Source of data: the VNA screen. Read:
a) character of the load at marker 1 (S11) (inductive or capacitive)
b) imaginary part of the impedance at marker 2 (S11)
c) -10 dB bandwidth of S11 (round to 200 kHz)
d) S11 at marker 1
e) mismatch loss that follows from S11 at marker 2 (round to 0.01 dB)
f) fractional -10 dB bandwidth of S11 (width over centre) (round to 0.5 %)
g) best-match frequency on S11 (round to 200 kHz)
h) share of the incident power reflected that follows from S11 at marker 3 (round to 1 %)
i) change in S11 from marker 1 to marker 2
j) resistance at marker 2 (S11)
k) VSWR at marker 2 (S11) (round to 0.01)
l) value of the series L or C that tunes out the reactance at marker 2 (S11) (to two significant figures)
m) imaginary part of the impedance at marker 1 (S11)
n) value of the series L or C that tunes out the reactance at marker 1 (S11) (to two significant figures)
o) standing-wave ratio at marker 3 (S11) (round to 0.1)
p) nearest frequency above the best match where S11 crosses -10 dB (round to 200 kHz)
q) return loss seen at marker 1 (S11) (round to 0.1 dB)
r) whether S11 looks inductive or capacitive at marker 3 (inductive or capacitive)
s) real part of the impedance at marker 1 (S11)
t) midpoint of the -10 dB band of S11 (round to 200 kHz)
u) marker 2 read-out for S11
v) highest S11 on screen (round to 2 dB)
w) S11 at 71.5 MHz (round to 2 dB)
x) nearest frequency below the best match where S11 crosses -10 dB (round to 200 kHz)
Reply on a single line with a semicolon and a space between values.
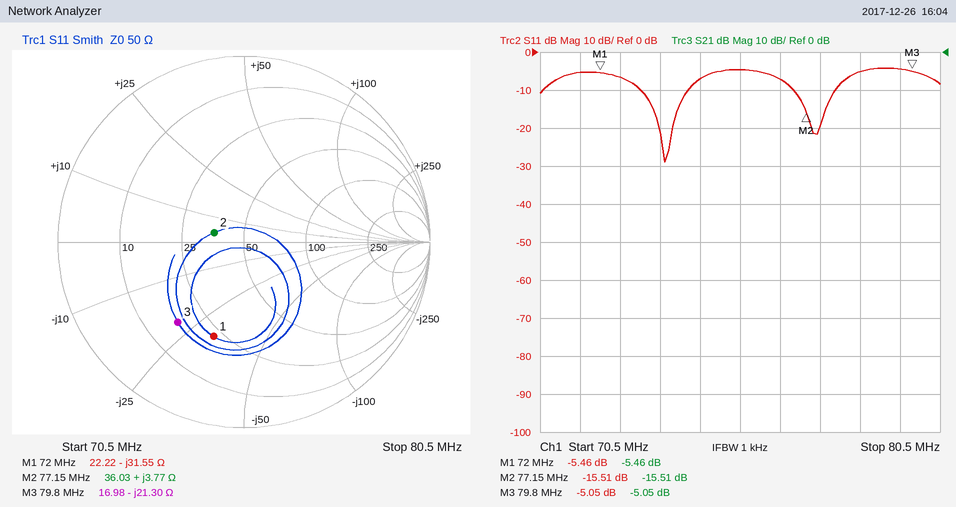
capacitive; +3.77 Ω; 1.2 MHz; -5.46 dB; 0.12 dB; 1.5 %; 73.6 MHz; 31 %; -10.05 dB; 36.03 Ω; 1.40; 550 pF; -31.55 Ω; 70 nH; 3.5; 74.2 MHz; 5.5 dB; capacitive; 22.22 Ω; 73.6 MHz; -15.51 dB; -4 dB; -6 dB; 73.0 MHz
